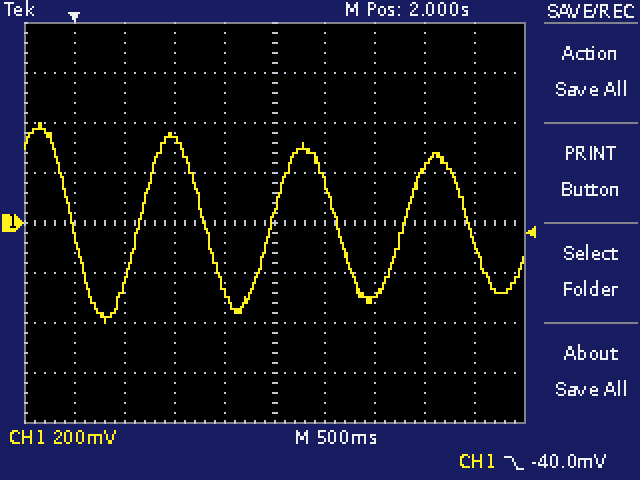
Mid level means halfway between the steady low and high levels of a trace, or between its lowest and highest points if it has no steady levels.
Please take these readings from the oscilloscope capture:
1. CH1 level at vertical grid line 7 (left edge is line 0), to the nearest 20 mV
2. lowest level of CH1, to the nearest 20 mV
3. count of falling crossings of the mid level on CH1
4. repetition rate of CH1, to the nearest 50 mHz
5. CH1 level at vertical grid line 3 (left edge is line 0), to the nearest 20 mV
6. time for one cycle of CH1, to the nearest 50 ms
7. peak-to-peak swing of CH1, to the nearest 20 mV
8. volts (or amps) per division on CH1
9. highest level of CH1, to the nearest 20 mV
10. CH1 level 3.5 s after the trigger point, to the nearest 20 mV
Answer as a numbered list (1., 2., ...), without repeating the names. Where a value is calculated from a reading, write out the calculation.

1. -300 mV
2. -400 mV
3. 4
4. 1 / 1.30 s ≈ 769 mHz, so 750 mHz to the nearest 50 mHz
5. 340 mV
6. 1.30 s
7. 400 mV − (-400 mV) = 800 mV
8. 200 mV
9. 400 mV
10. 220 mV
